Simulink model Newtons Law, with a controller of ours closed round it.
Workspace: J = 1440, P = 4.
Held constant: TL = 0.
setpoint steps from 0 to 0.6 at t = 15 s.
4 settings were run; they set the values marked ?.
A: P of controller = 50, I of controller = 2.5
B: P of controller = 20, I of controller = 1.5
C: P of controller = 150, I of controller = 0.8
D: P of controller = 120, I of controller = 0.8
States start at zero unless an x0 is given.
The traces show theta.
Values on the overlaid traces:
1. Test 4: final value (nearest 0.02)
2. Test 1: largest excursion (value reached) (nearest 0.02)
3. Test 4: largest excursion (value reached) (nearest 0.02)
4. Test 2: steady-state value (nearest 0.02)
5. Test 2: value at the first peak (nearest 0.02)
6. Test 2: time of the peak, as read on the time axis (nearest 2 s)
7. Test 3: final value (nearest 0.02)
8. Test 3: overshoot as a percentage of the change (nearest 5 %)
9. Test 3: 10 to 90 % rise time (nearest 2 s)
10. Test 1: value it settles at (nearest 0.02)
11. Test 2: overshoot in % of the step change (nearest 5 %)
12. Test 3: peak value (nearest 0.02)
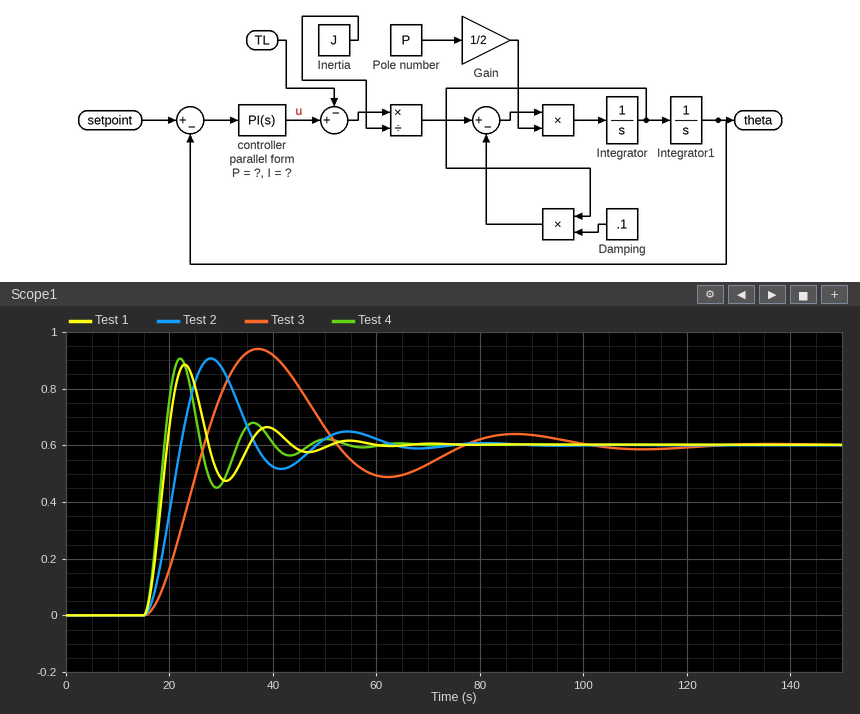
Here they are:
0.60
0.88
0.90
0.60
0.90
28 s
0.60
55 %
8 s
0.60
50 %
0.94
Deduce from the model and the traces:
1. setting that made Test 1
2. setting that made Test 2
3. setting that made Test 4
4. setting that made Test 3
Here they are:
D
A
C
B
